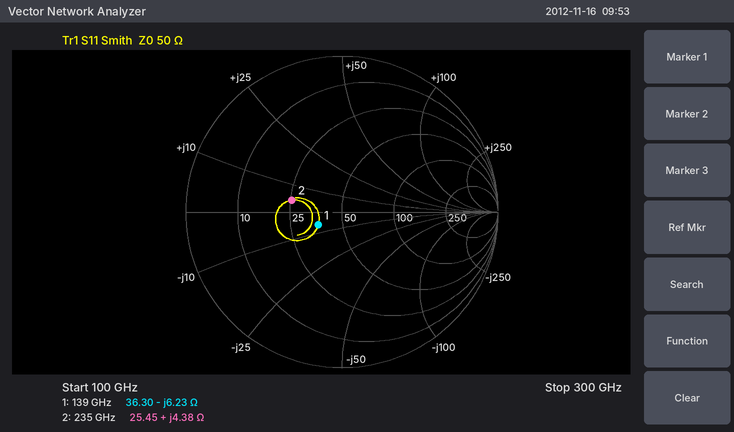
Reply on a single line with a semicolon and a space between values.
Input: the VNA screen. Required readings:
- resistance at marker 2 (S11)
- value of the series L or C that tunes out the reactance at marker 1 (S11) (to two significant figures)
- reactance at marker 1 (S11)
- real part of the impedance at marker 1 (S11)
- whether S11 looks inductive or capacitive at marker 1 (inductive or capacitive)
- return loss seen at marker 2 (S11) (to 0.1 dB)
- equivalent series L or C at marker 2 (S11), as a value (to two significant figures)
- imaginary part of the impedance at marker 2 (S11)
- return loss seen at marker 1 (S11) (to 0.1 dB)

25.45 Ω; 7.1 pH; -6.23 Ω; 36.30 Ω; capacitive; 9.6 dB; 3.0 pH; +4.38 Ω; 15.2 dB
